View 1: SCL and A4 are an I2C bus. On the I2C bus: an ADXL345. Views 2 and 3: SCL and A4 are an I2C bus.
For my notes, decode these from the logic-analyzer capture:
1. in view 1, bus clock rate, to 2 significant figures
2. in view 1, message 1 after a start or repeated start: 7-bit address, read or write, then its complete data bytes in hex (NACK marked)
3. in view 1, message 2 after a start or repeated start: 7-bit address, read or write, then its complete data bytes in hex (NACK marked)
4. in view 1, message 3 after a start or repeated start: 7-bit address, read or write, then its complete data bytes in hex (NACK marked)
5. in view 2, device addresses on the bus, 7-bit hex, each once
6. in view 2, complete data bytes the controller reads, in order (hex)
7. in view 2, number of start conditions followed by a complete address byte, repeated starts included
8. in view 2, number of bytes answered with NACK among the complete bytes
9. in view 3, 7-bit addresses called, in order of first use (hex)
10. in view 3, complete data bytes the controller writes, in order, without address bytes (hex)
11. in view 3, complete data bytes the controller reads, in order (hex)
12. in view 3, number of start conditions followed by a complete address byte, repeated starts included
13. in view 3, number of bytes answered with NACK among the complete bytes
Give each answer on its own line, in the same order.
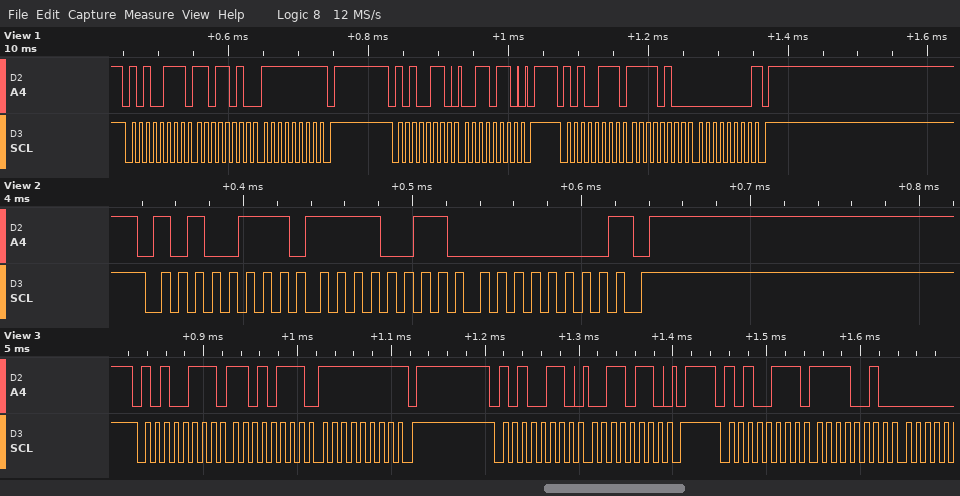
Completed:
100 kHz
0x53 read: DA FF NACK
0x53 write: 36
0x53 read: F4 00 NACK
0x53
F3 00
1
1
0x53
36
D7 FF F2
3
1
